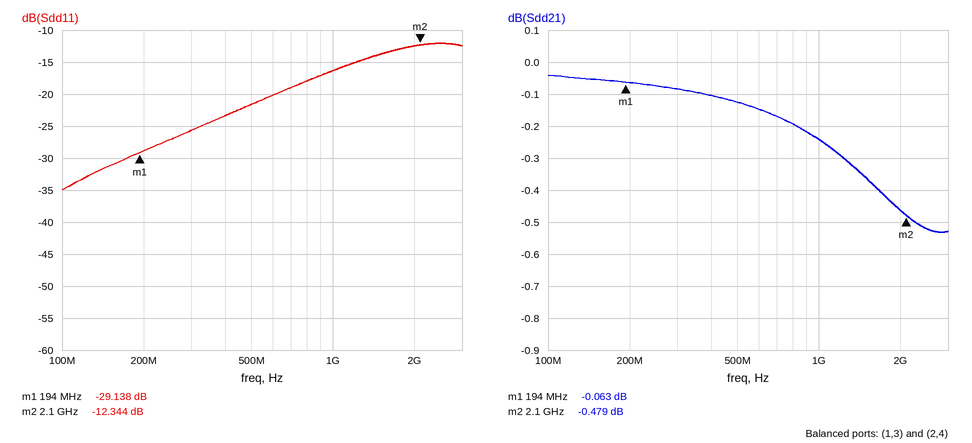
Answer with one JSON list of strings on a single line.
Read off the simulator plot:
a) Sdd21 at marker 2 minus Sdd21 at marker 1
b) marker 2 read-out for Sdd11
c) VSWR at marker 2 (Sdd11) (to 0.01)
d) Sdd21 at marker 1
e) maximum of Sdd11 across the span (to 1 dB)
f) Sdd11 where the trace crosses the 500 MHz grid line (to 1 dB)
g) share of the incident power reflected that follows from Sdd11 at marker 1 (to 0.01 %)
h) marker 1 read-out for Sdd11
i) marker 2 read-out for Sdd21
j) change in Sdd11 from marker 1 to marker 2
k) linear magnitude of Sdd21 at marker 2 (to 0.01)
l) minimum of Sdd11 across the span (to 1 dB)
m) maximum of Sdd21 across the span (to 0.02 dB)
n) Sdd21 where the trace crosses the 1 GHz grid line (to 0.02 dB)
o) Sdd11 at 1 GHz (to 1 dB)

["-0.416 dB", "-12.344 dB", "1.64", "-0.063 dB", "-12 dB", "-22 dB", "0.12 %", "-29.138 dB", "-0.479 dB", "16.794 dB", "0.95", "-35 dB", "-0.04 dB", "-0.24 dB", "-16 dB"]
